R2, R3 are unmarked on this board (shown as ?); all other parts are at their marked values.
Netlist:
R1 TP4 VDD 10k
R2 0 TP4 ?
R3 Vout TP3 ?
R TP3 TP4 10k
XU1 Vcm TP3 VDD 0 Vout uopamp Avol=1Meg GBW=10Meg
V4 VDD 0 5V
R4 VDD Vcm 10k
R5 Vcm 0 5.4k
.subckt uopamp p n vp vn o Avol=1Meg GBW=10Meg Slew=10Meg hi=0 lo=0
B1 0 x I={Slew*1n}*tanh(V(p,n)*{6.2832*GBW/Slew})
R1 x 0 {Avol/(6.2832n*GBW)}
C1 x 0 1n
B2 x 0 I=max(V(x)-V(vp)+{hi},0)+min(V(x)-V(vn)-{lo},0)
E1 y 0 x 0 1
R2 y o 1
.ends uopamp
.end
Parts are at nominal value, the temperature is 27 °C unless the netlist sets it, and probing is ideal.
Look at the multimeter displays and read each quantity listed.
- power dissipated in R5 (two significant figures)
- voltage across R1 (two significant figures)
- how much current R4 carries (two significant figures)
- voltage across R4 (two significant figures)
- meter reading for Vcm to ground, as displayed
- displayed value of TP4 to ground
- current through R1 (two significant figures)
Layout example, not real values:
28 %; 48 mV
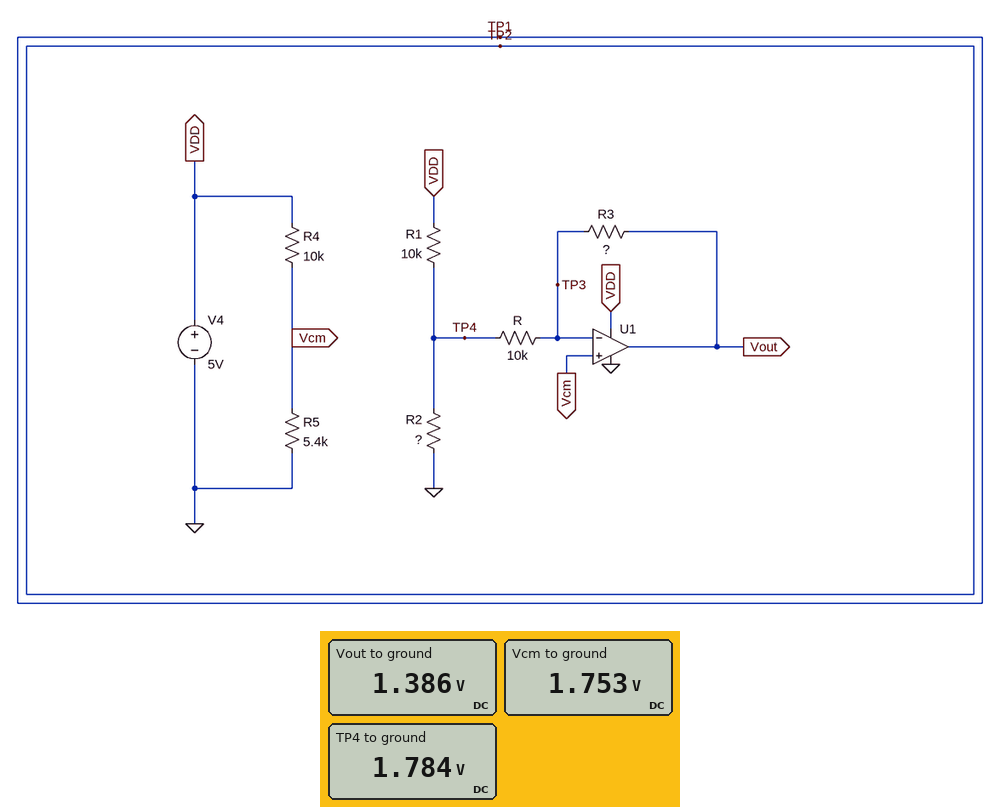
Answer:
570 µW; 3.2 V; 320 µA; 3.2 V; 1.753 V; 1.784 V; 320 µA
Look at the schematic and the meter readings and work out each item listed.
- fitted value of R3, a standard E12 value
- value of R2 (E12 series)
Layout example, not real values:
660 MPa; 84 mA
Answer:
120 kΩ; 5.6 kΩ
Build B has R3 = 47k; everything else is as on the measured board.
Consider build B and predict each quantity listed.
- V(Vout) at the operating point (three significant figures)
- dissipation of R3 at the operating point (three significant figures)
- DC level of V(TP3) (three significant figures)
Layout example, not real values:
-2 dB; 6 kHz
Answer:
1.61 V; 441 nW; 1.75 V
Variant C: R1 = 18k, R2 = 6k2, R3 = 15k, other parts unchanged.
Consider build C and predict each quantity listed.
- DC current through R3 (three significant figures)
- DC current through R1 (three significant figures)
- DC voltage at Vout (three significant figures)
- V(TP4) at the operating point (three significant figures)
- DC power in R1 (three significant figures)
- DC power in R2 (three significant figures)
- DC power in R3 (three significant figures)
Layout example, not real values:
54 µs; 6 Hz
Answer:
32.3 µA; 198 µA; 2.24 V; 1.43 V; 708 µW; 330 µW; 15.7 µW
